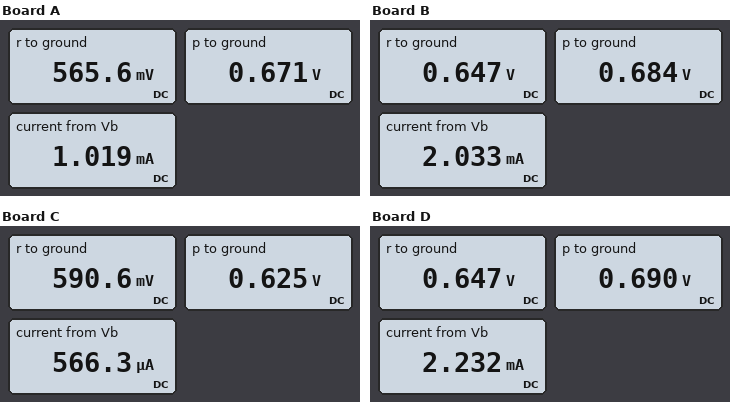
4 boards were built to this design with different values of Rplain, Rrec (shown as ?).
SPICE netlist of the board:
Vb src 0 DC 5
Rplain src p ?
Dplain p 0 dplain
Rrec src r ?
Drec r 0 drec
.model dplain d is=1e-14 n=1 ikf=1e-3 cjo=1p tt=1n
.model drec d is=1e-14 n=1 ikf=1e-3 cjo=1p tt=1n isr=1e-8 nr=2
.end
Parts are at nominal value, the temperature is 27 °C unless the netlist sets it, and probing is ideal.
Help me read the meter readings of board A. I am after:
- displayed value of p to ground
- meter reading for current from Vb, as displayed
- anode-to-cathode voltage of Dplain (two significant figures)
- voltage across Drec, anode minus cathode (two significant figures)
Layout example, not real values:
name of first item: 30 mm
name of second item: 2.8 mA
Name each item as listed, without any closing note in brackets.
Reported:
displayed value of p to ground: 0.671 V
meter reading for current from Vb, as displayed: 1.019 mA
anode-to-cathode voltage of Dplain: 670 mV
voltage across Drec, anode minus cathode: 570 mV
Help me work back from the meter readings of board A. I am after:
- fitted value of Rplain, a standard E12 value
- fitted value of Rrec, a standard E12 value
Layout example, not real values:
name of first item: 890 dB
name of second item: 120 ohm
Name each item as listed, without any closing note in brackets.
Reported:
fitted value of Rplain, a standard E12 value: 5.6 kΩ
fitted value of Rrec, a standard E12 value: 18 kΩ
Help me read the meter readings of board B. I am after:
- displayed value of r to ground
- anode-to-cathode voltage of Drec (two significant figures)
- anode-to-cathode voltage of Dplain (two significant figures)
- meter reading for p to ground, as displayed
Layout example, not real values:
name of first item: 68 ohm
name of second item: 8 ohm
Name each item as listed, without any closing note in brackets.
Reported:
displayed value of r to ground: 0.647 V
anode-to-cathode voltage of Drec: 650 mV
anode-to-cathode voltage of Dplain: 680 mV
meter reading for p to ground, as displayed: 0.684 V
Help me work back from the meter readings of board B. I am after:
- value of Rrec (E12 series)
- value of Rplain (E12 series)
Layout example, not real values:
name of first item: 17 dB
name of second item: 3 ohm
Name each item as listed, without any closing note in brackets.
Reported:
value of Rrec: 4.7 kΩ
value of Rplain: 3.9 kΩ
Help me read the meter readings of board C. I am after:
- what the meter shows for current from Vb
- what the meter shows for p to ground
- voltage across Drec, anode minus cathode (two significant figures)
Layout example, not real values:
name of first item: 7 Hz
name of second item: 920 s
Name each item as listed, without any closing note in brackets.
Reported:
what the meter shows for current from Vb: 566.3 µA
what the meter shows for p to ground: 0.625 V
voltage across Drec, anode minus cathode: 590 mV
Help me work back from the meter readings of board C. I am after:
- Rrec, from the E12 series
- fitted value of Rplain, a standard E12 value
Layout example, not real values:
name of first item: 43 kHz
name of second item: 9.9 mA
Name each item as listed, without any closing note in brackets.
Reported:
Rrec, from the E12 series: 12 kΩ
fitted value of Rplain, a standard E12 value: 22 kΩ
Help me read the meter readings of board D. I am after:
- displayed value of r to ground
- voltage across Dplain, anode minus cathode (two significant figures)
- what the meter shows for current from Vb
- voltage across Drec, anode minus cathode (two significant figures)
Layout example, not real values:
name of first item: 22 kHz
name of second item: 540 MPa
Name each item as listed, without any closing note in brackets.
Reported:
displayed value of r to ground: 0.647 V
voltage across Dplain, anode minus cathode: 690 mV
what the meter shows for current from Vb: 2.232 mA
voltage across Drec, anode minus cathode: 650 mV
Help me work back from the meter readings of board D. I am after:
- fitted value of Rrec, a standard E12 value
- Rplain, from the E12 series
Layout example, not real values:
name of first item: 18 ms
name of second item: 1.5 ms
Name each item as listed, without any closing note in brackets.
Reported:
fitted value of Rrec, a standard E12 value: 4.7 kΩ
Rplain, from the E12 series: 3.3 kΩ
